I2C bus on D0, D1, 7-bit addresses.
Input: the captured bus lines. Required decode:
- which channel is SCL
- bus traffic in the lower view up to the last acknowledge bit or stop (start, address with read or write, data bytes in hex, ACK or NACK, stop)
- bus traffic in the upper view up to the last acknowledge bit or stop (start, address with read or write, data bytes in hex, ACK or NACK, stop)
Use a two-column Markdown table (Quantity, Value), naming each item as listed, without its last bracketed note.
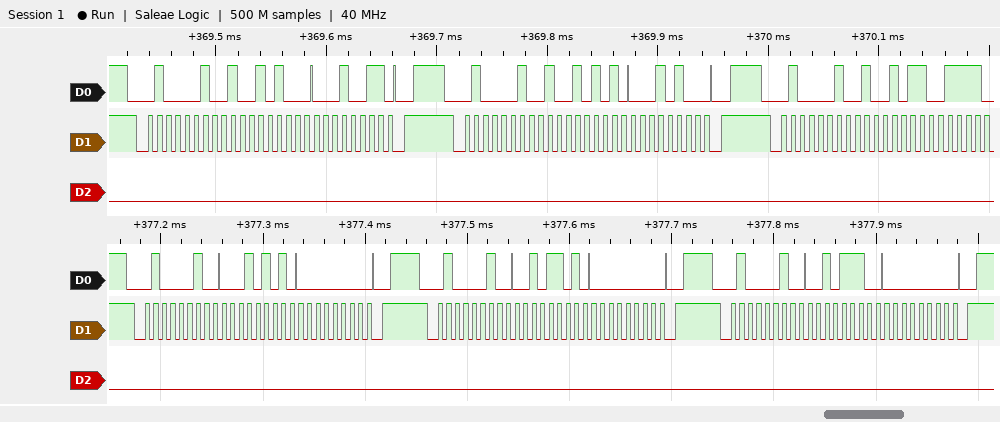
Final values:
| Quantity | Value |
|---|---|
| which channel is SCL | D1 |
| bus traffic in the lower view up to the last acknowledge bit or stop | start, address 21 write ACK, 15 ACK, 00 ACK, stop, start, address 21 write ACK, 2D ACK, 00 ACK, stop, start, address 21 write ACK, 2E ACK, 00 ACK, stop |
| bus traffic in the upper view up to the last acknowledge bit or stop | start, address 21 write ACK, 94 ACK, 13 ACK, stop, start, address 21 write ACK, 95 ACK, 14 ACK, stop, start, address 21 write ACK, 96 ACK |
